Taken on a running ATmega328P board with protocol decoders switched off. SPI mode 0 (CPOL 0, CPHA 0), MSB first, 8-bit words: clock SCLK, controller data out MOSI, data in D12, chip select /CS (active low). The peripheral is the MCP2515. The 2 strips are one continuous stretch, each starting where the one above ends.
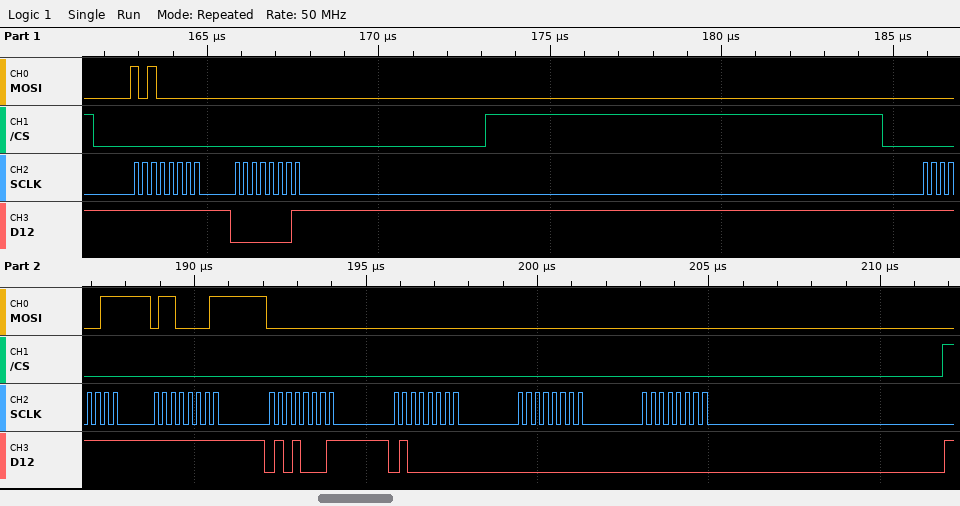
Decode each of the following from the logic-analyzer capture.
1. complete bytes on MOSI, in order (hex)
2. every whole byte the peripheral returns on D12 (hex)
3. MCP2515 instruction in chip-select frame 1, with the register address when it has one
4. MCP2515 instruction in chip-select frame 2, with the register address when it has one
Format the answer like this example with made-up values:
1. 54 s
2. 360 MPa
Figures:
1. A0 00 03 61 00 00 00 00
2. FF 01 FF FF 51 40 00 00
3. READ STATUS
4. READ 0x61
